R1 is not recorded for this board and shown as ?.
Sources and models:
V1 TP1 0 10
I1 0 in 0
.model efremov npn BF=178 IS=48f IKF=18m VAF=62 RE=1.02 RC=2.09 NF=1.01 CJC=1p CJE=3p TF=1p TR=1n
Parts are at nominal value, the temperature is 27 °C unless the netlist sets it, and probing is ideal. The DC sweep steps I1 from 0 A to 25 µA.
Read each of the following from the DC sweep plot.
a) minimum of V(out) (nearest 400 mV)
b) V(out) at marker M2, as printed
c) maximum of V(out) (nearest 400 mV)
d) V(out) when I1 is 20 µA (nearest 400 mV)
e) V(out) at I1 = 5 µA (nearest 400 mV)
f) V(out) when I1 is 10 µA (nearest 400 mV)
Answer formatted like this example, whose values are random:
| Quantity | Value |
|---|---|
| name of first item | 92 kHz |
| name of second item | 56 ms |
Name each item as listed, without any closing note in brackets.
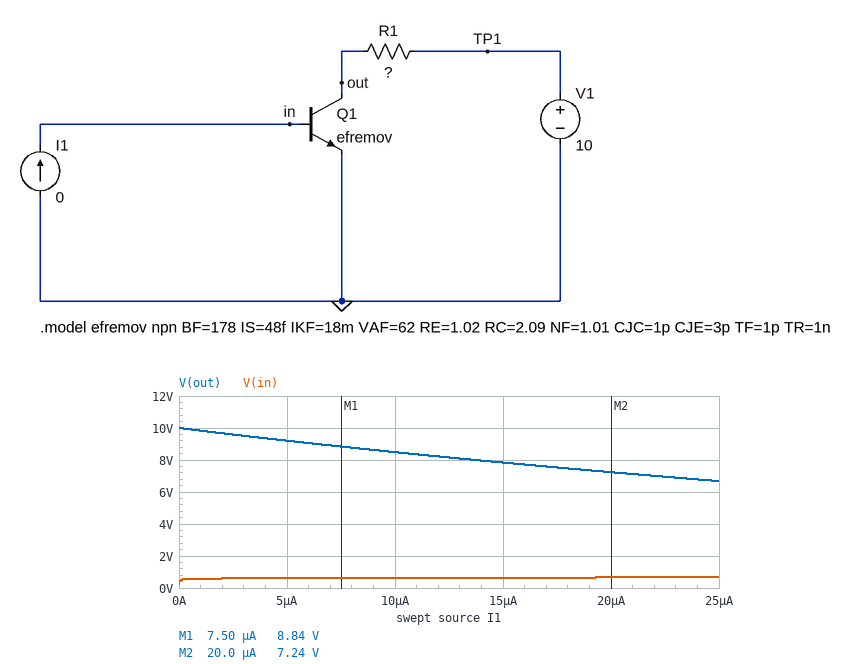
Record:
| Quantity | Value |
|---|---|
| minimum of V(out) | 6.8 V |
| V(out) at marker M2, as printed | 7.24 V |
| maximum of V(out) | 10.0 V |
| V(out) when I1 is 20 µA | 7.2 V |
| V(out) at I1 = 5 µA | 9.2 V |
| V(out) when I1 is 10 µA | 8.4 V |
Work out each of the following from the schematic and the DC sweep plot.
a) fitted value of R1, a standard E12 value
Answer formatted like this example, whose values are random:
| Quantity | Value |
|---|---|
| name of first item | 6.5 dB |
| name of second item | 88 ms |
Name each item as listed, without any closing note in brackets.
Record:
| Quantity | Value |
|---|---|
| fitted value of R1, a standard E12 value | 820 Ω |
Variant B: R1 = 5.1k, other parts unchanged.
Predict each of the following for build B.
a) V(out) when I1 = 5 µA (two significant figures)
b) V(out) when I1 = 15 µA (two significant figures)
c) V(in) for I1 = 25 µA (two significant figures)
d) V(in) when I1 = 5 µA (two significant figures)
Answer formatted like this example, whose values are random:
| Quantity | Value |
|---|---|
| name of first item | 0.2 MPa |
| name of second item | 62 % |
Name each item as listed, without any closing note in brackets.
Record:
| Quantity | Value |
|---|---|
| V(out) when I1 = 5 µA | 5.3 V |
| V(out) when I1 = 15 µA | 180 mV |
| V(in) for I1 = 25 µA | 640 mV |
| V(in) when I1 = 5 µA | 620 mV |
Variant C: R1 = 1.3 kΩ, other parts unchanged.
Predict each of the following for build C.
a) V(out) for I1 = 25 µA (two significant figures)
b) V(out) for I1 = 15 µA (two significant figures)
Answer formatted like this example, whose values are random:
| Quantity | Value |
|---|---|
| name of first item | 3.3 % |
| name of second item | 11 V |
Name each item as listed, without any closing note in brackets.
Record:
| Quantity | Value |
|---|---|
| V(out) for I1 = 25 µA | 4.9 V |
| V(out) for I1 = 15 µA | 6.6 V |
